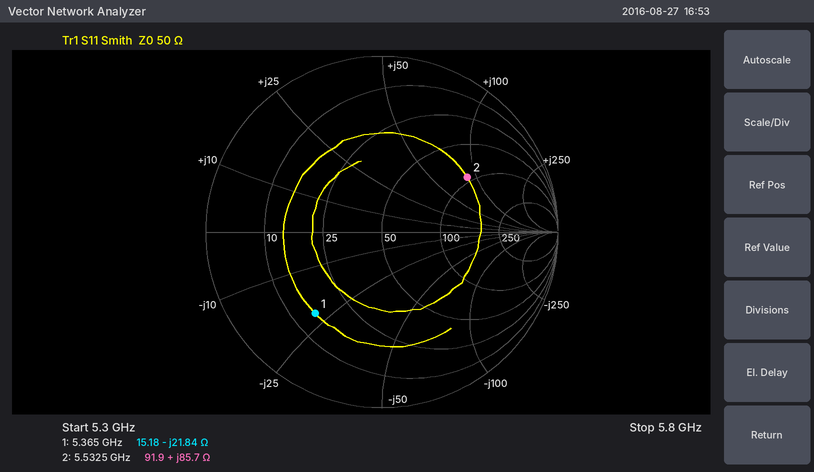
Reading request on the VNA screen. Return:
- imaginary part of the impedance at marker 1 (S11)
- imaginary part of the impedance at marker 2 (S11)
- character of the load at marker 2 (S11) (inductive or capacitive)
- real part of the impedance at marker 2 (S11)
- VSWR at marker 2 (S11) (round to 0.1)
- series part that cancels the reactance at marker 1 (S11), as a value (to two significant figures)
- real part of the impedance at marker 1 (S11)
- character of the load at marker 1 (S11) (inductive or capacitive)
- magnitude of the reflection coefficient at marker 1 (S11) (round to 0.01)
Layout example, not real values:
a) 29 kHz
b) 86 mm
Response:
a) -21.84 Ω
b) +85.7 Ω
c) inductive
d) 91.9 Ω
e) 3.7
f) 650 pH
g) 15.18 Ω
h) capacitive
i) 0.60
